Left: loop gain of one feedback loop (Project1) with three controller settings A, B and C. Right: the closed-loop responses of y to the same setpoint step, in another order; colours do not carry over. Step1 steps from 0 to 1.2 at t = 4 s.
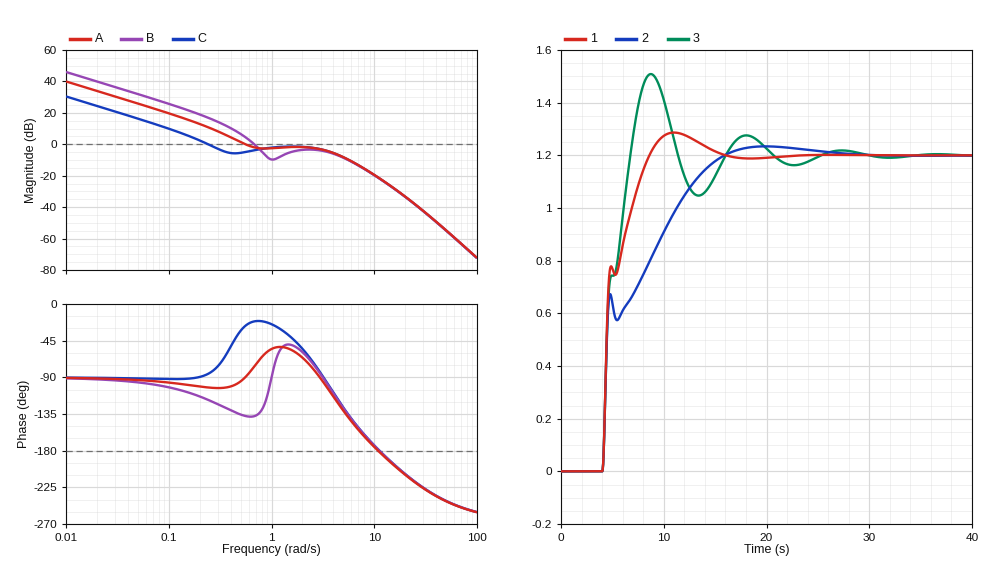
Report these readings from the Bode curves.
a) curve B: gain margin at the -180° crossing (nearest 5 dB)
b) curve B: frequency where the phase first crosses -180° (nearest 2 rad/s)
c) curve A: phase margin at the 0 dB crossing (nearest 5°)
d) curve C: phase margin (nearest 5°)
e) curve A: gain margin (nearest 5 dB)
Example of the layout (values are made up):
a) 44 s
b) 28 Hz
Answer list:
a) 20 dB
b) 12 rad/s
c) 90°
d) 95°
e) 20 dB
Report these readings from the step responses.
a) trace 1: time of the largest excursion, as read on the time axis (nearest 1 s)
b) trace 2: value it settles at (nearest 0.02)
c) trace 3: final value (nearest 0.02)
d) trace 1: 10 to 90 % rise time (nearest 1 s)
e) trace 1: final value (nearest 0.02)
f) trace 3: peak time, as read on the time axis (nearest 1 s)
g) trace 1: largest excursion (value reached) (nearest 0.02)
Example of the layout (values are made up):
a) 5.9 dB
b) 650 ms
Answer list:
a) 11 s
b) 1.20
c) 1.20
d) 3 s
e) 1.20
f) 9 s
g) 1.28
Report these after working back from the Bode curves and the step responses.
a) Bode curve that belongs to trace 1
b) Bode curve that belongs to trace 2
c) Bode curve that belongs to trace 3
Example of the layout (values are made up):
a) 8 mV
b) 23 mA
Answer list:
a) A
b) C
c) B
